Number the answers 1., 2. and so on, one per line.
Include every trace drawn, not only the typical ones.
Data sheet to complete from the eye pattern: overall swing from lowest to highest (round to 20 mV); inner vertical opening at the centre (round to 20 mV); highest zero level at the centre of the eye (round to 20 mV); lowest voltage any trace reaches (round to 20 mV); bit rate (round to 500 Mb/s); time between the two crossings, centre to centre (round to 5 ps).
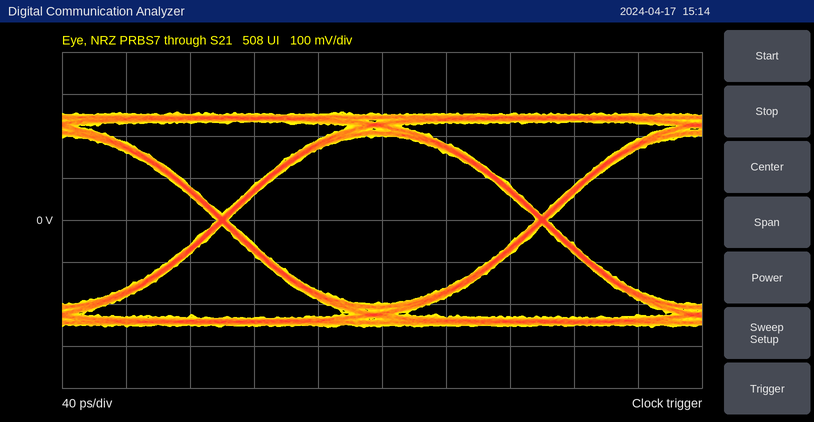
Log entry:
1. 520 mV
2. 400 mV
3. -200 mV
4. -260 mV
5. 5.0 Gb/s
6. 200 ps
